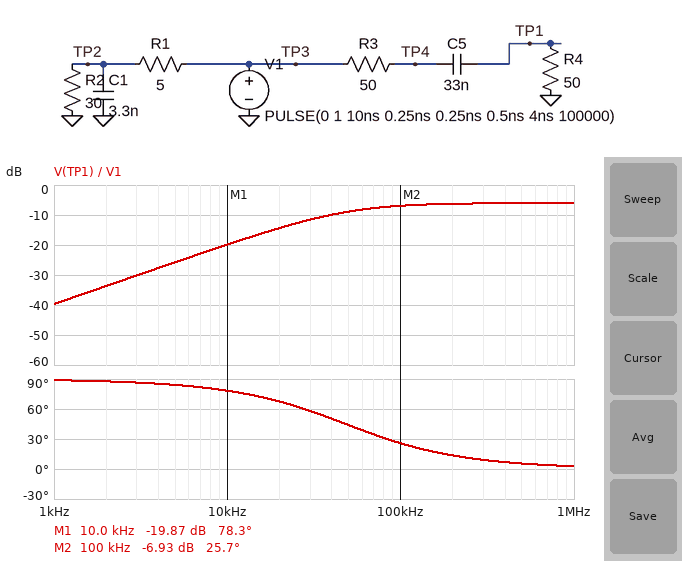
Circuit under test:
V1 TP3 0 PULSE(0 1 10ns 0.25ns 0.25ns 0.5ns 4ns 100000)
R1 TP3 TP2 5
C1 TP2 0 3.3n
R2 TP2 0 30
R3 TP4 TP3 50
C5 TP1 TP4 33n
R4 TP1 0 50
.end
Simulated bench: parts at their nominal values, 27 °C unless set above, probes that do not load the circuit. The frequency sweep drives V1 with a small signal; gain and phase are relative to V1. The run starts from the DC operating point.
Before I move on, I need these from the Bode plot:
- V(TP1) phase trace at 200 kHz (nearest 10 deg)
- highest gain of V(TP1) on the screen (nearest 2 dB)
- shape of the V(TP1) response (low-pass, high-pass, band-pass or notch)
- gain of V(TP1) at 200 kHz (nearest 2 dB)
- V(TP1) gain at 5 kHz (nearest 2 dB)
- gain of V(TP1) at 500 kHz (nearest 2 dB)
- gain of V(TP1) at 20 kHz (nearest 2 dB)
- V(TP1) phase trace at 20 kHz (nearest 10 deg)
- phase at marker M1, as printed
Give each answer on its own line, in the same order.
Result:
10 deg
-6 dB
high-pass
-6 dB
-26 dB
-6 dB
-14 dB
70 deg
78.3 deg
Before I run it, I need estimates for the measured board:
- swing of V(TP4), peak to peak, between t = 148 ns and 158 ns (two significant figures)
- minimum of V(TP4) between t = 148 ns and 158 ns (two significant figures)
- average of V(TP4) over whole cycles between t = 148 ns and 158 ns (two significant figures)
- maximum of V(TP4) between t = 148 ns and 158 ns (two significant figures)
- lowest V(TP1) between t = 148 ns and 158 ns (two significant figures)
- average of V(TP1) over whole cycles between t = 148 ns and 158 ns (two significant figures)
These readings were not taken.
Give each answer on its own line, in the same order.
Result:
500 mV
3.9 mV
98 mV
500 mV
-4.1 mV
90 mV
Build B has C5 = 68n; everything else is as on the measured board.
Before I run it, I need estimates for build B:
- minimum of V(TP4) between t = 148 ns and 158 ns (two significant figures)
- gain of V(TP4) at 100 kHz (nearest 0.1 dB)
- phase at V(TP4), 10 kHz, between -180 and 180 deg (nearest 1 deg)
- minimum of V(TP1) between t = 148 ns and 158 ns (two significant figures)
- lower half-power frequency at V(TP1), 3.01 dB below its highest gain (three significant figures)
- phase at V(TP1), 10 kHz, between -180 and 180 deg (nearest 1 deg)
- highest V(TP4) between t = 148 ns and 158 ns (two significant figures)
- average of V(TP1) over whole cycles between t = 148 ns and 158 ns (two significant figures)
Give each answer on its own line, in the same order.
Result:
1.9 mV
-5.4 dB
-11 deg
-2.0 mV
23.4 kHz
67 deg
500 mV
92 mV
